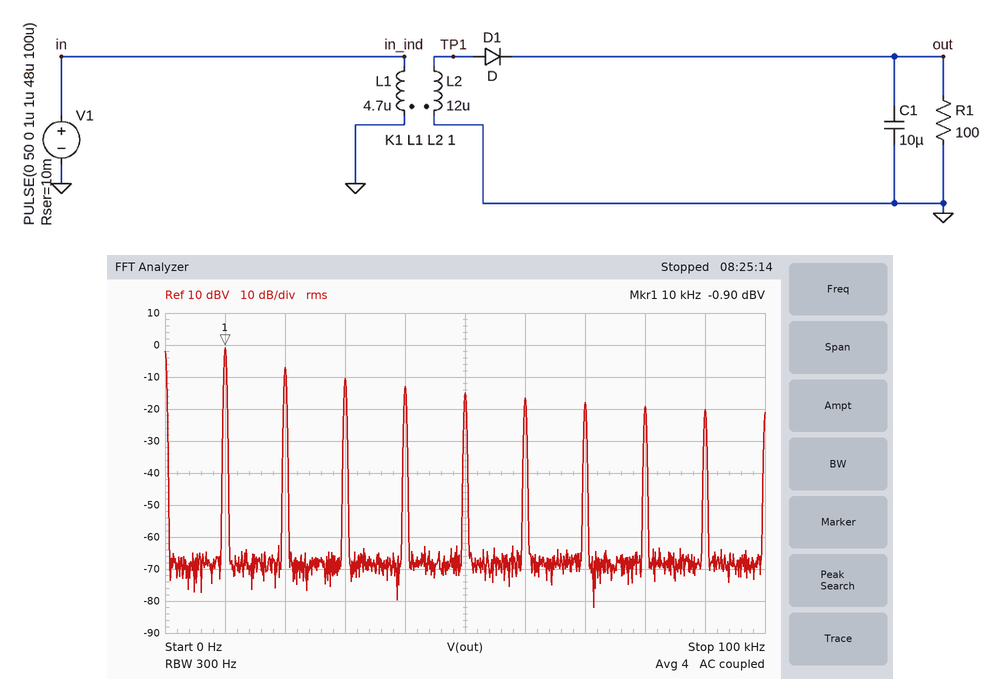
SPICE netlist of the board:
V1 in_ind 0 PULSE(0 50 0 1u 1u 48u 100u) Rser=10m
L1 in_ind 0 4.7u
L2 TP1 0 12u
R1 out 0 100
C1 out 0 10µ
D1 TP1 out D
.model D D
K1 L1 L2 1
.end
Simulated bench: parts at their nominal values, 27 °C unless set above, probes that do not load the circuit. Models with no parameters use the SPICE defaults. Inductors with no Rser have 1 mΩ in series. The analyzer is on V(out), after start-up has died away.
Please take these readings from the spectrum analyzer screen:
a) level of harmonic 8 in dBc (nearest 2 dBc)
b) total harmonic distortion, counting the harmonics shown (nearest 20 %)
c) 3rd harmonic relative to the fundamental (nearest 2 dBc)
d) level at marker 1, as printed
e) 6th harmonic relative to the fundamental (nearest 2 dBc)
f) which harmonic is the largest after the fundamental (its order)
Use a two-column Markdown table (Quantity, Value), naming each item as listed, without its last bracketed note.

| Quantity | Value |
|---|---|
| level of harmonic 8 in dBc | -18 dBc |
| total harmonic distortion, counting the harmonics shown | 80 % |
| 3rd harmonic relative to the fundamental | -10 dBc |
| level at marker 1, as printed | -0.90 dBV |
| 6th harmonic relative to the fundamental | -16 dBc |
| which harmonic is the largest after the fundamental | 2 |
